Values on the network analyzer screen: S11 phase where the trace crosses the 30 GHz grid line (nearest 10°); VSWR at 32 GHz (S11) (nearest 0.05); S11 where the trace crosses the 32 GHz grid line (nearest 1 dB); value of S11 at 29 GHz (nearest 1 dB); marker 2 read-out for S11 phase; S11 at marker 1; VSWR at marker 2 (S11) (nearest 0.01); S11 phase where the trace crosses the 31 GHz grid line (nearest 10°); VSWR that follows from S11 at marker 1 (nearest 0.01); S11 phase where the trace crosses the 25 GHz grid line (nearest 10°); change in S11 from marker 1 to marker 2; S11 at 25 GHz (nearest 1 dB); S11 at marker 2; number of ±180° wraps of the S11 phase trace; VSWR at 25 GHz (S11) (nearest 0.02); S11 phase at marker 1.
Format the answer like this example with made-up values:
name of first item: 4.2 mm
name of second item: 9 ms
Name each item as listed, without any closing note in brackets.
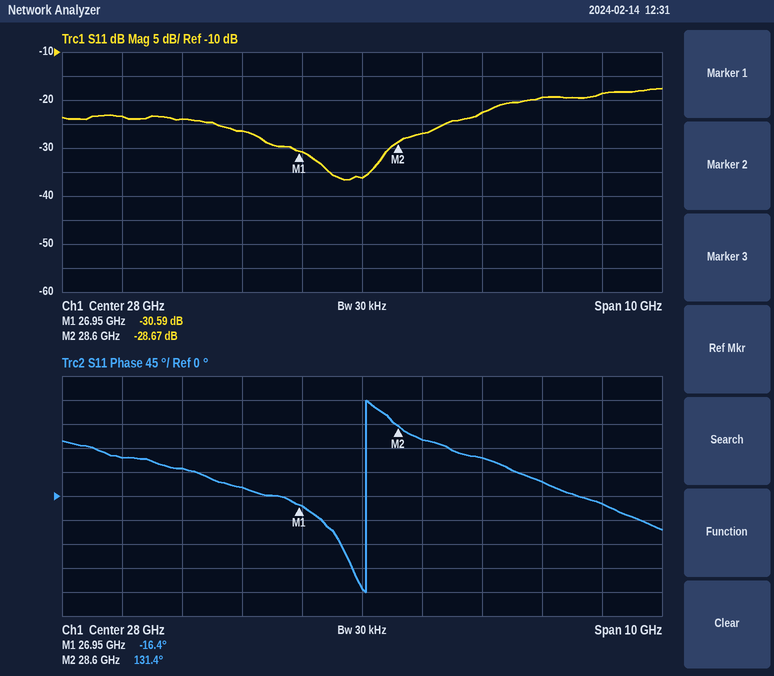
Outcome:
S11 phase where the trace crosses the 30 GHz grid line: 70°
VSWR at 32 GHz (S11): 1.25
S11 where the trace crosses the 32 GHz grid line: -19 dB
value of S11 at 29 GHz: -27 dB
marker 2 read-out for S11 phase: 131.4°
S11 at marker 1: -30.59 dB
VSWR at marker 2 (S11): 1.08
S11 phase where the trace crosses the 31 GHz grid line: 30°
VSWR that follows from S11 at marker 1: 1.06
S11 phase where the trace crosses the 25 GHz grid line: 50°
change in S11 from marker 1 to marker 2: 1.92 dB
S11 at 25 GHz: -24 dB
S11 at marker 2: -28.67 dB
number of ±180° wraps of the S11 phase trace: 1
VSWR at 25 GHz (S11): 1.14
S11 phase at marker 1: -16.4°
